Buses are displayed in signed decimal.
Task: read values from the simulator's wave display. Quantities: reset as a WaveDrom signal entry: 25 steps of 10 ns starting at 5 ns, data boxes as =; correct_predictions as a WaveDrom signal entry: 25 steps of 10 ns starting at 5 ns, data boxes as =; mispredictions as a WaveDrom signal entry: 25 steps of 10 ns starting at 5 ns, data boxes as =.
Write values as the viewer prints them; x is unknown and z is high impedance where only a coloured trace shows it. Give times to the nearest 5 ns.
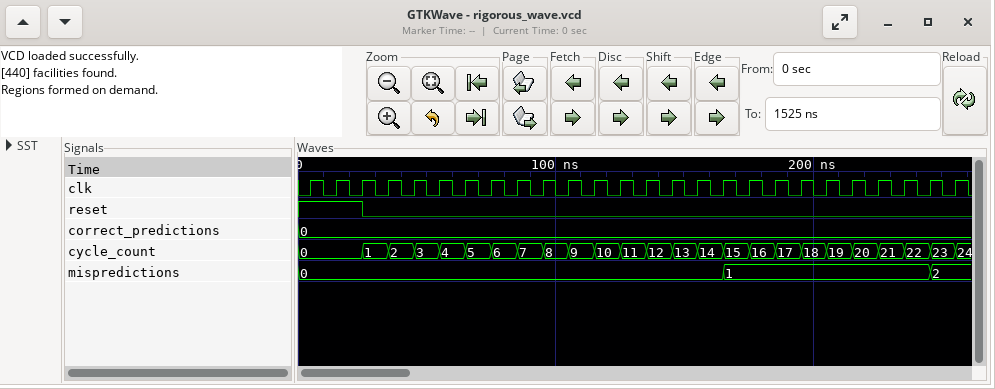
{name: 'reset', wave: '1.0......................'}
{name: 'correct_predictions', wave: '=........................', data: '0'}
{name: 'mispredictions', wave: '=...............=.......=', data: '0 1 2'}
